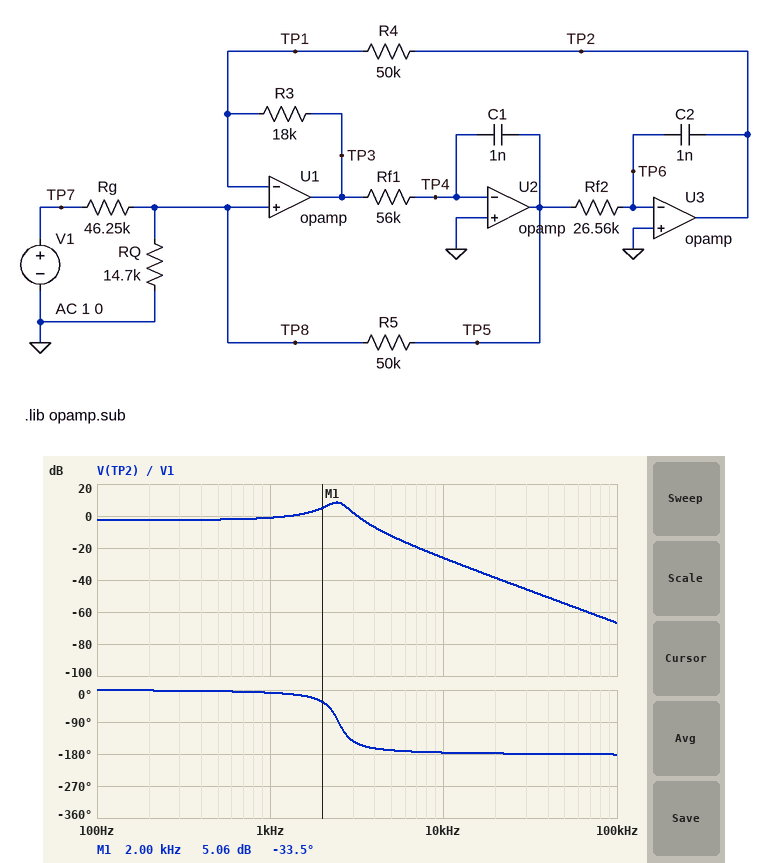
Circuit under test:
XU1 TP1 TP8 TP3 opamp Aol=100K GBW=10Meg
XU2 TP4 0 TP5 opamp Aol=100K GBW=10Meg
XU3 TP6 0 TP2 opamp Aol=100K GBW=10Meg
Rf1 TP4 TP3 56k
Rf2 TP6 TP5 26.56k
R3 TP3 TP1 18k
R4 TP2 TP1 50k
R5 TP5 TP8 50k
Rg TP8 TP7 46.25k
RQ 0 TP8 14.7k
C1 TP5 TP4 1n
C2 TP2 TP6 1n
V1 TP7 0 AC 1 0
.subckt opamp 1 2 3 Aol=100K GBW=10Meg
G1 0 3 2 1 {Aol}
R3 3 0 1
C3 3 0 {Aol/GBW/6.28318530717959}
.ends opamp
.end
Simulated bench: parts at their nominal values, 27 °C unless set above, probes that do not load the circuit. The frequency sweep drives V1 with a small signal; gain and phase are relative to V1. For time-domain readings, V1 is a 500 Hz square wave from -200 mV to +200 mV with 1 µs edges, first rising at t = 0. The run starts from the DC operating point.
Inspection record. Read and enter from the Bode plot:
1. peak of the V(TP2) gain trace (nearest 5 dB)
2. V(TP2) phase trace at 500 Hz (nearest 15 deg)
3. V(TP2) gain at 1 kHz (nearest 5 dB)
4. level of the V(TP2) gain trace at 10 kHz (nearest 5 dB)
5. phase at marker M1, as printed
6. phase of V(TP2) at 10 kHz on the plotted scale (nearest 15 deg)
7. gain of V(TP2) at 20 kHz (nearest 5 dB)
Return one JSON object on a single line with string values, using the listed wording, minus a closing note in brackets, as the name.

{"peak of the V(TP2) gain trace": "10 dB", "V(TP2) phase trace at 500 Hz": "0 deg", "V(TP2) gain at 1 kHz": "0 dB", "level of the V(TP2) gain trace at 10 kHz": "-25 dB", "phase at marker M1, as printed": "-33.5 deg", "phase of V(TP2) at 10 kHz on the plotted scale": "-180 deg", "gain of V(TP2) at 20 kHz": "-40 dB"}
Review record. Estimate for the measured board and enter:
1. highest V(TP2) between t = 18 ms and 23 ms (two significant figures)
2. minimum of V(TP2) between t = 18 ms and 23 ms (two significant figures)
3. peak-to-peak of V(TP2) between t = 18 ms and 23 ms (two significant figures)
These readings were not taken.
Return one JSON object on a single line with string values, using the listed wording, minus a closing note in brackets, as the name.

{"highest V(TP2) between t = 18 ms and 23 ms": "360 mV", "minimum of V(TP2) between t = 18 ms and 23 ms": "-360 mV", "peak-to-peak of V(TP2) between t = 18 ms and 23 ms": "720 mV"}
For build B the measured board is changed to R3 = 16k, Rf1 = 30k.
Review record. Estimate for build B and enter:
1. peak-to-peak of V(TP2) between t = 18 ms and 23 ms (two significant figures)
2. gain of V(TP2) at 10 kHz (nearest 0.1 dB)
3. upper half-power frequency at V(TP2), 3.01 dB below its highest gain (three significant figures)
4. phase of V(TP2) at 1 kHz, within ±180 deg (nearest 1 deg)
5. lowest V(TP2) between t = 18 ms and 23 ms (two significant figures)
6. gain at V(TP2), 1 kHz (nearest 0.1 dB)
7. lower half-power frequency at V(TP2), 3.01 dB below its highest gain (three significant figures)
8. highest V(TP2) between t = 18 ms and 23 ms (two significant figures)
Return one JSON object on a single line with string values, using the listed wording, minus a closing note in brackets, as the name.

{"peak-to-peak of V(TP2) between t = 18 ms and 23 ms": "660 mV", "gain of V(TP2) at 10 kHz": "-20.8 dB", "upper half-power frequency at V(TP2), 3.01 dB below its highest gain": "3.65 kHz", "phase of V(TP2) at 1 kHz, within ±180 deg": "-8 deg", "lowest V(TP2) between t = 18 ms and 23 ms": "-330 mV", "gain at V(TP2), 1 kHz": "-1.0 dB", "lower half-power frequency at V(TP2), 3.01 dB below its highest gain": "2.32 kHz", "highest V(TP2) between t = 18 ms and 23 ms": "330 mV"}
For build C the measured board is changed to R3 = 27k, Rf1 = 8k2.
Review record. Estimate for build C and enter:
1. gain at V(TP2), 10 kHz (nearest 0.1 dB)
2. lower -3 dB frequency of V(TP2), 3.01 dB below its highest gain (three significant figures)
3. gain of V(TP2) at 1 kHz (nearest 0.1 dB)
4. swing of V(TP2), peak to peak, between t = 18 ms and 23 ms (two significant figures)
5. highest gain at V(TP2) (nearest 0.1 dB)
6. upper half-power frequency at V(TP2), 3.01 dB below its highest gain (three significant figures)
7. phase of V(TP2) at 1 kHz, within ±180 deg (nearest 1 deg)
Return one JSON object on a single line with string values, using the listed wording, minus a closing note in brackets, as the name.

{"gain at V(TP2), 10 kHz": "-5.4 dB", "lower -3 dB frequency of V(TP2), 3.01 dB below its highest gain": "2.76 kHz", "gain of V(TP2) at 1 kHz": "-4.9 dB", "swing of V(TP2), peak to peak, between t = 18 ms and 23 ms": "370 mV", "highest gain at V(TP2)": "-1.2 dB", "upper half-power frequency at V(TP2), 3.01 dB below its highest gain": "9.40 kHz", "phase of V(TP2) at 1 kHz, within ±180 deg": "-5 deg"}
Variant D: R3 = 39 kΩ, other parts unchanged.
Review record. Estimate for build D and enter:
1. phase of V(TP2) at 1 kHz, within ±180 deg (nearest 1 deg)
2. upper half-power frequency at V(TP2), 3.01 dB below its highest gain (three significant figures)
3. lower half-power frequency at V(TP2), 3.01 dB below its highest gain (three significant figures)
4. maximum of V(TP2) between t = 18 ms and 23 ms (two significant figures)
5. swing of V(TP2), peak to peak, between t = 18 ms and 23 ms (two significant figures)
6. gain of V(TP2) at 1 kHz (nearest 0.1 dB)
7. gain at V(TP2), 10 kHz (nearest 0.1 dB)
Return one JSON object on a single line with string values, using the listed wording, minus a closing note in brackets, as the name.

{"phase of V(TP2) at 1 kHz, within ±180 deg": "-4 deg", "upper half-power frequency at V(TP2), 3.01 dB below its highest gain": "4.02 kHz", "lower half-power frequency at V(TP2), 3.01 dB below its highest gain": "3.09 kHz", "maximum of V(TP2) between t = 18 ms and 23 ms": "220 mV", "swing of V(TP2), peak to peak, between t = 18 ms and 23 ms": "430 mV", "gain of V(TP2) at 1 kHz": "-6.3 dB", "gain at V(TP2), 10 kHz": "-23.3 dB"}
